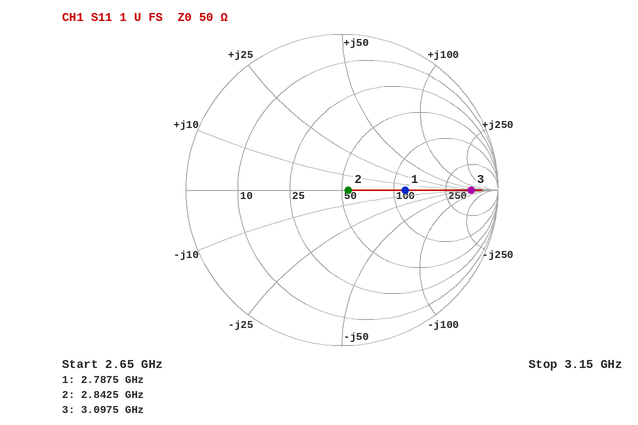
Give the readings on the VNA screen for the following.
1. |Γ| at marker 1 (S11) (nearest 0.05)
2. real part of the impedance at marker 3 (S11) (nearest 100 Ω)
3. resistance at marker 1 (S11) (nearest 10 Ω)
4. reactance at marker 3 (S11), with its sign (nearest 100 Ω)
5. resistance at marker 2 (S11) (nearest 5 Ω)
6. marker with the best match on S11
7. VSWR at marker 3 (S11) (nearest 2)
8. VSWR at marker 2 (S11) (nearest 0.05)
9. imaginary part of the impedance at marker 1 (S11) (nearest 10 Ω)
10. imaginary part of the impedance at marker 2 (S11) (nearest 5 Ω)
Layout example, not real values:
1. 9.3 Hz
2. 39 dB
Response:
1. 0.40
2. 500 Ω
3. 120 Ω
4. 0 Ω
5. 55 Ω
6. marker 2
7. 10
8. 1.10
9. 0 Ω
10. 0 Ω
